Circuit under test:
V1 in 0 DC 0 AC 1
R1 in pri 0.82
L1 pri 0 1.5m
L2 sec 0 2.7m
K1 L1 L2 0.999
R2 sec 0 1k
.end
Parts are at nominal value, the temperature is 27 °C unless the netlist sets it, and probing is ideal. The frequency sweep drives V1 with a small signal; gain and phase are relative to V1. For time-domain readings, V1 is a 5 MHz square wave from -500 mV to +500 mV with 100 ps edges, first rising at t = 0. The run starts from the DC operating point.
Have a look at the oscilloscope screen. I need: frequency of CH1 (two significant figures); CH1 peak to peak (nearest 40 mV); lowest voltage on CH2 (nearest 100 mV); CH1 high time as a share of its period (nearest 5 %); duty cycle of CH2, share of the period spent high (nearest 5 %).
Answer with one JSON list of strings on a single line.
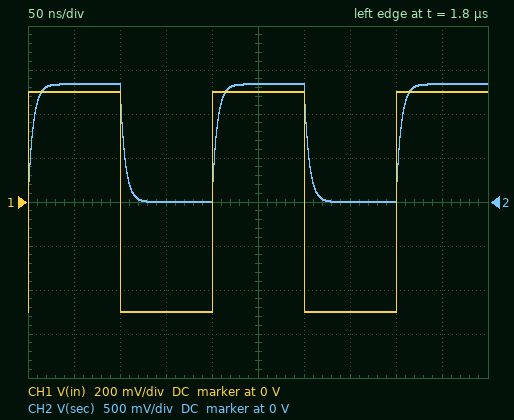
["5.0 MHz", "1.00 V", "0 V", "50 %", "50 %"]
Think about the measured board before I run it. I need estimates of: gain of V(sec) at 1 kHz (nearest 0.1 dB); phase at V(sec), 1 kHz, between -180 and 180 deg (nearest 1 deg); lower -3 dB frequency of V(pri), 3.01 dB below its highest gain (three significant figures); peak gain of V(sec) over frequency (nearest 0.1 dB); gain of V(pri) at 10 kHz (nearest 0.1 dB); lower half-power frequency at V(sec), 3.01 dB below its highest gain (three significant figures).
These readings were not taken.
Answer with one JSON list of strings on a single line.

["2.5 dB", "5 deg", "86.9 Hz", "2.5 dB", "0 dB", "86.9 Hz"]
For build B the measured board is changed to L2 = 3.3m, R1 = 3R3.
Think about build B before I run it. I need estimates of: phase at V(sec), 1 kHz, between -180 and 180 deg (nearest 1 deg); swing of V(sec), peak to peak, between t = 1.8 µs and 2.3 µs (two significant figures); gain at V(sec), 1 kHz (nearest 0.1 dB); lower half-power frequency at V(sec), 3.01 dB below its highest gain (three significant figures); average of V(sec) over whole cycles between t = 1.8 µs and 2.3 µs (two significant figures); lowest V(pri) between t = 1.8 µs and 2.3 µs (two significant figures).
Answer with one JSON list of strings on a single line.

["19 deg", "1.5 V", "2.9 dB", "348 Hz", "730 mV", "-9.5 mV"]
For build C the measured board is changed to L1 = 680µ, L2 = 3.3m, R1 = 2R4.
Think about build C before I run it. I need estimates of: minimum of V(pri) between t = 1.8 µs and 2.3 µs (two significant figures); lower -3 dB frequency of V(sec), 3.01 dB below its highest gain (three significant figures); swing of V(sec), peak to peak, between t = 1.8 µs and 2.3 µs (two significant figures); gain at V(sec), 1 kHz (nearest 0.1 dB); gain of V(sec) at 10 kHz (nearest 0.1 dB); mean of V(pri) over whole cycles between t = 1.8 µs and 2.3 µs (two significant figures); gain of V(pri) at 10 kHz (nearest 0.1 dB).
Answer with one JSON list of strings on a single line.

["-15 mV", "555 Hz", "2.2 V", "5.6 dB", "6.7 dB", "490 mV", "-0.1 dB"]
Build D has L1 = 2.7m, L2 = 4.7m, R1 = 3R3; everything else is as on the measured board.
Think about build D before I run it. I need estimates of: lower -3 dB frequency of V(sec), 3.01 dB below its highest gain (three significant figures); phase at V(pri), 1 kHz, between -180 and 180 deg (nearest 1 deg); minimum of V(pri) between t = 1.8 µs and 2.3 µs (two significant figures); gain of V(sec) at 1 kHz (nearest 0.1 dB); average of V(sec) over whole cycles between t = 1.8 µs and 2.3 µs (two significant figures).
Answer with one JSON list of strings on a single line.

["193 Hz", "11 deg", "-7.0 mV", "2.2 dB", "650 mV"]
